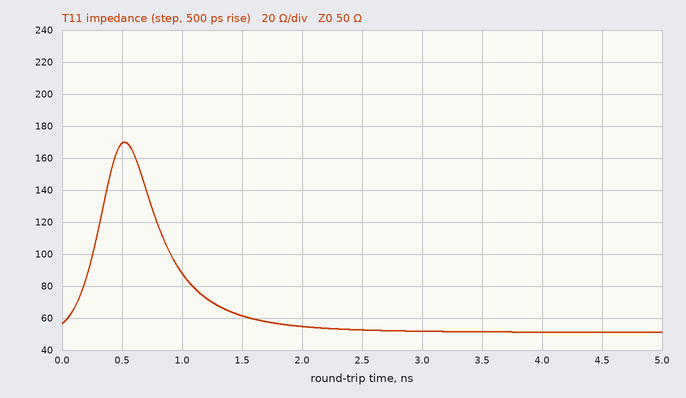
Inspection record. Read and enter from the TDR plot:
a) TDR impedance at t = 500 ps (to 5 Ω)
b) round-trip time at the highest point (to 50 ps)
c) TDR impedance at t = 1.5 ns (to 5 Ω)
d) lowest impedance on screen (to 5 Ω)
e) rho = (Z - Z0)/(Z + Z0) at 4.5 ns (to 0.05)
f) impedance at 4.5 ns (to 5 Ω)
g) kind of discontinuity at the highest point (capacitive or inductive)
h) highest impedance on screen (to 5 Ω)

170 Ω
500 ps
60 Ω
50 Ω
0.00
50 Ω
inductive
170 Ω
